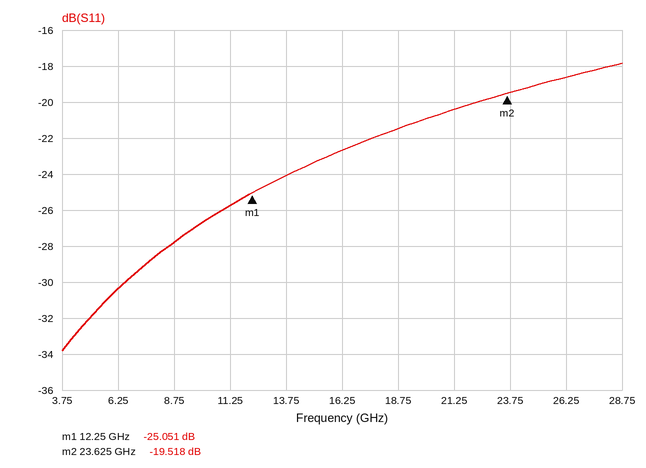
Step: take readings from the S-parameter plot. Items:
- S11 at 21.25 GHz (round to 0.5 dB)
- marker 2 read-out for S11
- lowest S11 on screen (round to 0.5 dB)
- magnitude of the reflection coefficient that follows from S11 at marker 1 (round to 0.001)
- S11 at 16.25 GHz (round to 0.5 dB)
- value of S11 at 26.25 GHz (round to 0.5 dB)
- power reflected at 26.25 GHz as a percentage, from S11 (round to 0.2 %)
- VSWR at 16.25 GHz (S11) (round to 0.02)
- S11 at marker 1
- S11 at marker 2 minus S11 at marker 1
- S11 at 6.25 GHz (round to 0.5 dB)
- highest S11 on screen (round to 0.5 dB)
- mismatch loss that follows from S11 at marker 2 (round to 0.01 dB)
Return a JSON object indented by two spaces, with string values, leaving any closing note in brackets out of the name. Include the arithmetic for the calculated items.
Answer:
{
  "S11 at 21.25 GHz": "-20.5 dB",
  "marker 2 read-out for S11": "-19.518 dB",
  "lowest S11 on screen": "-34.0 dB",
  "magnitude of the reflection coefficient that follows from S11 at marker 1": "10^(-25.051/20) ≈ 0.056",
  "S11 at 16.25 GHz": "-22.5 dB",
  "value of S11 at 26.25 GHz": "-18.5 dB",
  "power reflected at 26.25 GHz as a percentage, from S11": "10^(-18.5/10) ≈ 1.4 %",
  "VSWR at 16.25 GHz (S11)": "|Γ| = 10^(-22.5/20) = 0.0750; VSWR = (1 + 0.0750)/(1 − 0.0750) ≈ 1.16",
  "S11 at marker 1": "-25.051 dB",
  "S11 at marker 2 minus S11 at marker 1": "-19.518 − (-25.051) = 5.533 dB",
  "S11 at 6.25 GHz": "-30.5 dB",
  "highest S11 on screen": "-18.0 dB",
  "mismatch loss that follows from S11 at marker 2": "−10 log10(1 − 10^(-19.518/10)) ≈ 0.05 dB"
}
